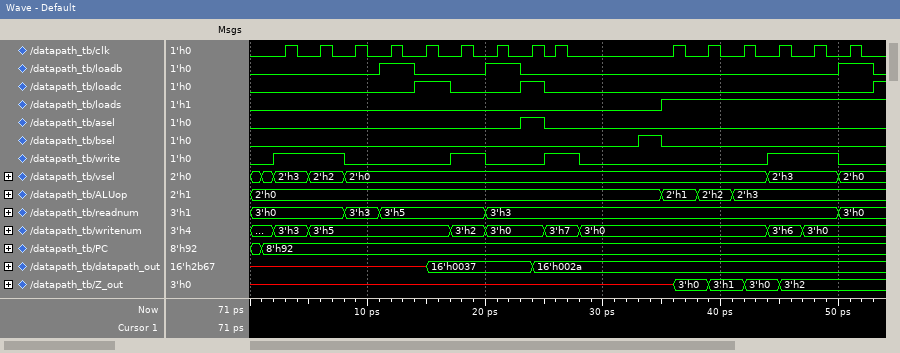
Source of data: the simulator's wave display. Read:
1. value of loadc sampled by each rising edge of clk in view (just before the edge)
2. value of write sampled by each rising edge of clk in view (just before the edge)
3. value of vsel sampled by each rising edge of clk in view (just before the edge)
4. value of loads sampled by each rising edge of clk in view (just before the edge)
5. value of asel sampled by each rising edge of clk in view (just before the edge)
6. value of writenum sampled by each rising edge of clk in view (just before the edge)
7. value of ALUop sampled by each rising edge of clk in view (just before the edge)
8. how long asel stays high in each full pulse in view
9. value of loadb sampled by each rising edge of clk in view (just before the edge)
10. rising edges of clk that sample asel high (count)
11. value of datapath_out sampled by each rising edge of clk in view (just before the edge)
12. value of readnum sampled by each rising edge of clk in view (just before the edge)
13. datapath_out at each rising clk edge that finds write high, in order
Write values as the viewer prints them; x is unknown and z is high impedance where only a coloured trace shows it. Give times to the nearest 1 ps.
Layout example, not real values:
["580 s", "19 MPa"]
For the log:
["0 0 0 0 1 0 0 1 0 0 0 0 0 0 0", "1 1 0 0 0 1 0 0 1 0 0 0 1 1 0", "2'h3, 2'h2, 2'h0, 2'h0, 2'h0, 2'h0, 2'h0, 2'h0, 2'h0, 2'h0, 2'h0, 2'h0, 2'h3, 2'h3, 2'h0", "0 0 0 0 0 0 0 0 0 1 1 1 1 1 1", "0 0 0 0 0 0 0 1 0 0 0 0 0 0 0", "3'h3, 3'h5, 3'h5, 3'h5, 3'h5, 3'h2, 3'h0, 3'h0, 3'h7, 3'h0, 3'h0, 3'h0, 3'h6, 3'h0, 3'h0", "2'h0, 2'h0, 2'h0, 2'h0, 2'h0, 2'h0, 2'h0, 2'h0, 2'h0, 2'h1, 2'h2, 2'h3, 2'h3, 2'h3, 2'h3", "2 ps", "0 0 0 1 0 0 1 0 0 0 0 0 0 0 1", "1", "x, x, x, x, x, 16'h0037, 16'h0037, 16'h0037, 16'h002a, 16'h002a, 16'h002a, 16'h002a, 16'h002a, 16'h002a, 16'h002a", "3'h0, 3'h0, 3'h3, 3'h5, 3'h5, 3'h5, 3'h3, 3'h3, 3'h3, 3'h3, 3'h3, 3'h3, 3'h3, 3'h3, 3'h0", "x, x, 16'h0037, 16'h002a, 16'h002a, 16'h002a"]
